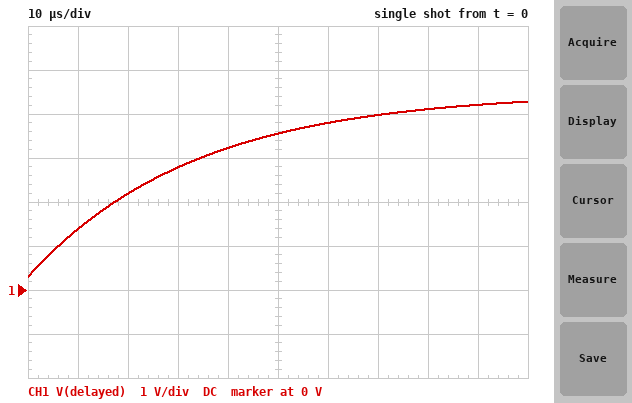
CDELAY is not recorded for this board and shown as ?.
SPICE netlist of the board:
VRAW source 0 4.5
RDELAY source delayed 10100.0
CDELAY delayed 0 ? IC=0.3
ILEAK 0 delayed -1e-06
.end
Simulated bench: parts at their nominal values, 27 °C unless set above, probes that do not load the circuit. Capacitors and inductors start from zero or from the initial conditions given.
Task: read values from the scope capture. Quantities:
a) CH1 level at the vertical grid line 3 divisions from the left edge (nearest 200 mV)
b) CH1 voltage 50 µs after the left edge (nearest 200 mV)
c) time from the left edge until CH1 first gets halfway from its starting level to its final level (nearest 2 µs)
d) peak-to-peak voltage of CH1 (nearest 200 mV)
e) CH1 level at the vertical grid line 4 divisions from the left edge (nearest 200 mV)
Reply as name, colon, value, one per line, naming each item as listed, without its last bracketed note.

CH1 level at the vertical grid line 3 divisions from the left edge: 2.8 V
CH1 voltage 50 µs after the left edge: 3.6 V
time from the left edge until CH1 first gets halfway from its starting level to its final level: 22 µs
peak-to-peak voltage of CH1: 4.0 V
CH1 level at the vertical grid line 4 divisions from the left edge: 3.2 V
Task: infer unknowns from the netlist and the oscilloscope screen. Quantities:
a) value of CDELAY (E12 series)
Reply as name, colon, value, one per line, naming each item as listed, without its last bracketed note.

value of CDELAY: 3.3 nF
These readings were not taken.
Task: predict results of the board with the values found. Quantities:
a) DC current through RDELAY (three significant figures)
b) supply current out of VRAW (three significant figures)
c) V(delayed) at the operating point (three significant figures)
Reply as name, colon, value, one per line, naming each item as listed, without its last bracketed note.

DC current through RDELAY: 1.00 µA
supply current out of VRAW: 1.00 µA
V(delayed) at the operating point: 4.49 V
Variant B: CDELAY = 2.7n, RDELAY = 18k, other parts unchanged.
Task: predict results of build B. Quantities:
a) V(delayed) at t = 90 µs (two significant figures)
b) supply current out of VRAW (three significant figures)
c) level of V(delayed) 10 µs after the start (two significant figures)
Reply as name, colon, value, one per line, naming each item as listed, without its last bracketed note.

V(delayed) at t = 90 µs: 3.8 V
supply current out of VRAW: 1.00 µA
level of V(delayed) 10 µs after the start: 1.1 V
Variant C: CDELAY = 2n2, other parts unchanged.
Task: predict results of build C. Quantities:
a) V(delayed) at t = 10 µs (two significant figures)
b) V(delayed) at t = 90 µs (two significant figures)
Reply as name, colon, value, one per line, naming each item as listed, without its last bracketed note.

V(delayed) at t = 10 µs: 1.8 V
V(delayed) at t = 90 µs: 4.4 V
